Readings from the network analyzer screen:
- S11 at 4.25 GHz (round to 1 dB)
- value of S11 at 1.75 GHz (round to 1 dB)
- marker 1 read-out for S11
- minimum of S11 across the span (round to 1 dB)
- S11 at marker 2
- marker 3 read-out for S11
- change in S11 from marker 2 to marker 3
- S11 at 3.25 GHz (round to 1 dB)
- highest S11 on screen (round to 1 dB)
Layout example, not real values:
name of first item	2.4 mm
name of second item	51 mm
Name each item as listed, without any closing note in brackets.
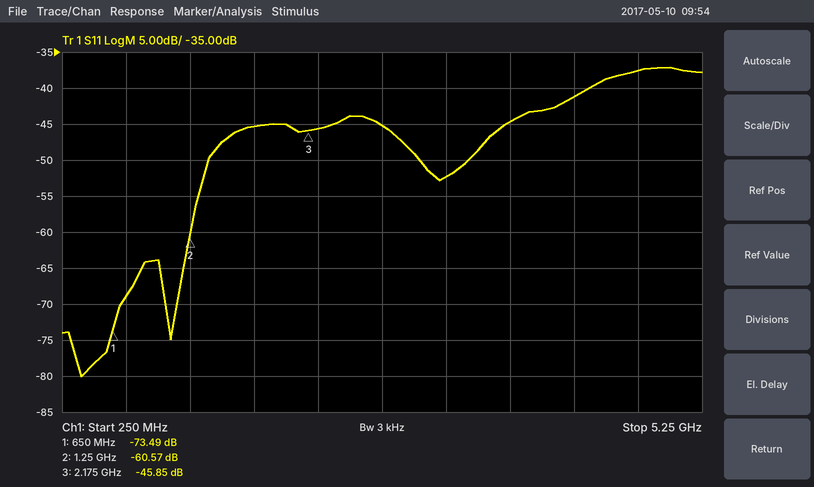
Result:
S11 at 4.25 GHz	-41 dB
value of S11 at 1.75 GHz	-45 dB
marker 1 read-out for S11	-73.49 dB
minimum of S11 across the span	-80 dB
S11 at marker 2	-60.57 dB
marker 3 read-out for S11	-45.85 dB
change in S11 from marker 2 to marker 3	14.72 dB
S11 at 3.25 GHz	-52 dB
highest S11 on screen	-37 dB
